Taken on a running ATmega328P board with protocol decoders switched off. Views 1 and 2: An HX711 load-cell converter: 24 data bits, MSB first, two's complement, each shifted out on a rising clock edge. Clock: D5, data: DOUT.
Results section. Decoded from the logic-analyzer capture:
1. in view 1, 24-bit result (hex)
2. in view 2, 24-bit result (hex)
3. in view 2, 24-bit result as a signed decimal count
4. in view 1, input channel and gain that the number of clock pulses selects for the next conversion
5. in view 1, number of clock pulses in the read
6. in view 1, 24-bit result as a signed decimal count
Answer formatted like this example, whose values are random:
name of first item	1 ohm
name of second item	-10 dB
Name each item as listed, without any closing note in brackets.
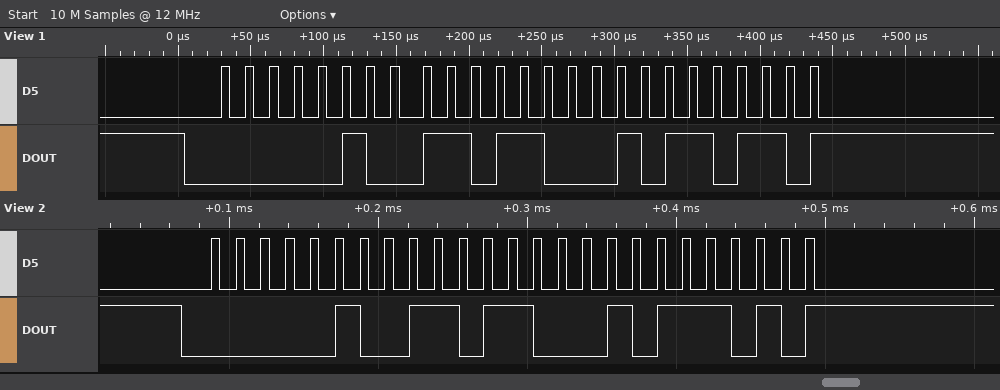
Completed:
in view 1, 24-bit result	0x04D8B6
in view 2, 24-bit result	0x04D8BA
in view 2, 24-bit result as a signed decimal count	317626
in view 1, input channel and gain that the number of clock pulses selects for the next conversion	channel A, gain 128
in view 1, number of clock pulses in the read	25
in view 1, 24-bit result as a signed decimal count	317622
